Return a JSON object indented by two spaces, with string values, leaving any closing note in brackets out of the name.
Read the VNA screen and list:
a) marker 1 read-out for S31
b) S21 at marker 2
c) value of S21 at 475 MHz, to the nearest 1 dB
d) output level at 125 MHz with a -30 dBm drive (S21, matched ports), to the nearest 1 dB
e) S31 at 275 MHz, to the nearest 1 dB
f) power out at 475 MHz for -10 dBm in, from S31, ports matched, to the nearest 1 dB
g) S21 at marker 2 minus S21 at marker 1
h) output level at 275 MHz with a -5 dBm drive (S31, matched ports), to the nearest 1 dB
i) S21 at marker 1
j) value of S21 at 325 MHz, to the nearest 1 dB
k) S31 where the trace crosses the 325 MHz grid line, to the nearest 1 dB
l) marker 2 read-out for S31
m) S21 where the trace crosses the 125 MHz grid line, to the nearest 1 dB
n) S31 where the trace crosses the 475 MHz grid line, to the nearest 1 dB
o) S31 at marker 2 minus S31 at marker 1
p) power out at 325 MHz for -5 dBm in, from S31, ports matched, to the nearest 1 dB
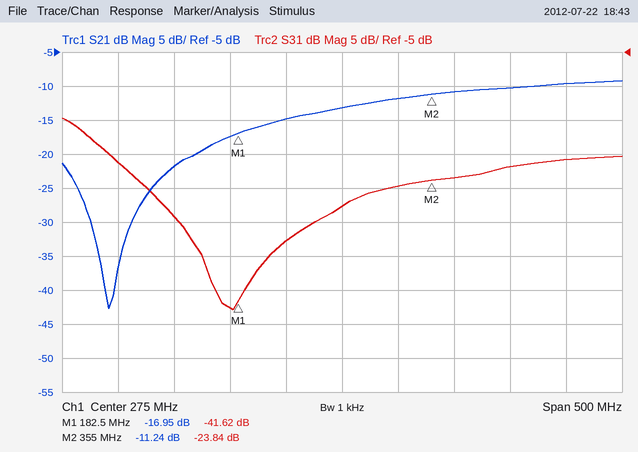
{
  "marker 1 read-out for S31": "-41.62 dB",
  "S21 at marker 2": "-11.24 dB",
  "value of S21 at 475 MHz, to the nearest 1 dB": "-10 dB",
  "output level at 125 MHz with a -30 dBm drive (S21, matched ports), to the nearest 1 dB": "-52 dBm",
  "S31 at 275 MHz, to the nearest 1 dB": "-28 dB",
  "power out at 475 MHz for -10 dBm in, from S31, ports matched, to the nearest 1 dB": "-31 dBm",
  "S21 at marker 2 minus S21 at marker 1": "5.71 dB",
  "output level at 275 MHz with a -5 dBm drive (S31, matched ports), to the nearest 1 dB": "-33 dBm",
  "S21 at marker 1": "-16.95 dB",
  "value of S21 at 325 MHz, to the nearest 1 dB": "-12 dB",
  "S31 where the trace crosses the 325 MHz grid line, to the nearest 1 dB": "-25 dB",
  "marker 2 read-out for S31": "-23.84 dB",
  "S21 where the trace crosses the 125 MHz grid line, to the nearest 1 dB": "-22 dB",
  "S31 where the trace crosses the 475 MHz grid line, to the nearest 1 dB": "-21 dB",
  "S31 at marker 2 minus S31 at marker 1": "17.78 dB",
  "power out at 325 MHz for -5 dBm in, from S31, ports matched, to the nearest 1 dB": "-30 dBm"
}
